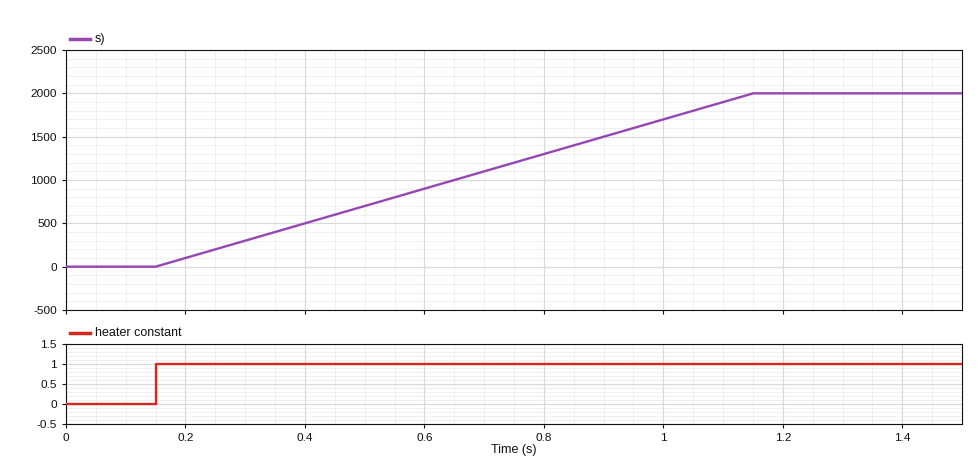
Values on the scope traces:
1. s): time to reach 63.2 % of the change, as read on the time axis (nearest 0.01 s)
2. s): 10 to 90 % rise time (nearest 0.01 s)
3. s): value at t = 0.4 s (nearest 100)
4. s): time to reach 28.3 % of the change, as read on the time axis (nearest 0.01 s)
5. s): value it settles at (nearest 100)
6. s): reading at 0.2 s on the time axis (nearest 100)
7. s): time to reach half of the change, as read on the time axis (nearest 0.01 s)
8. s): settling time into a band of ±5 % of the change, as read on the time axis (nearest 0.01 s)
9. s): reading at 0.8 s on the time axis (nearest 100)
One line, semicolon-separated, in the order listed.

0.78 s; 0.80 s; 500; 0.43 s; 2000; 100; 0.65 s; 1.10 s; 1300
